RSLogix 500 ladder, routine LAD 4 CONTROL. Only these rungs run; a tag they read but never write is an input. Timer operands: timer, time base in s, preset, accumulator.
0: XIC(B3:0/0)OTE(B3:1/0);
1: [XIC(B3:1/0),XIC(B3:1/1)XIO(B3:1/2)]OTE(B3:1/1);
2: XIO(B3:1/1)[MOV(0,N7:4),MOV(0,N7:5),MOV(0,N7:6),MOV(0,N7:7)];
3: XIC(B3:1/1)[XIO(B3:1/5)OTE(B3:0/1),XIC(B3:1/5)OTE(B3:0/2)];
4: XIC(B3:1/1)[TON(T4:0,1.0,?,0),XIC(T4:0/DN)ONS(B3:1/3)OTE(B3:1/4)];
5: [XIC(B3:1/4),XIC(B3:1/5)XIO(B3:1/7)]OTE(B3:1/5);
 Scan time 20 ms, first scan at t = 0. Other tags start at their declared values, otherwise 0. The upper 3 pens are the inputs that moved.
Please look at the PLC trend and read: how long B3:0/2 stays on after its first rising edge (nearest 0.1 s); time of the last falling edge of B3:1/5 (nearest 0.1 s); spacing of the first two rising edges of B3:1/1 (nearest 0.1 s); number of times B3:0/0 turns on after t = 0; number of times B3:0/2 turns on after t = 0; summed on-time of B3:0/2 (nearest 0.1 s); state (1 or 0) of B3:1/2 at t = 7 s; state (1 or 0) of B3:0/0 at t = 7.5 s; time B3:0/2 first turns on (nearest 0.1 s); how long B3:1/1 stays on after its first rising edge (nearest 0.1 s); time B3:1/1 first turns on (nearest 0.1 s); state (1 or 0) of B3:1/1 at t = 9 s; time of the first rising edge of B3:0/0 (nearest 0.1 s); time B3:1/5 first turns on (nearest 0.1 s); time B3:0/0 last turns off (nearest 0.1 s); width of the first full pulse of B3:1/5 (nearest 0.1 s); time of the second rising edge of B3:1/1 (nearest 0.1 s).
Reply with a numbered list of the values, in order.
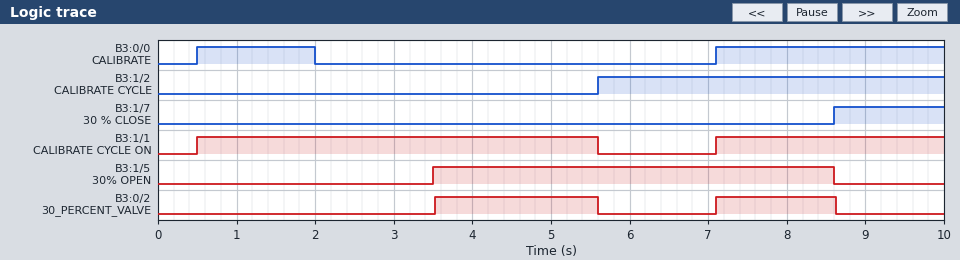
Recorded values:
1. 2.1 s
2. 8.6 s
3. 6.6 s
4. 2
5. 2
6. 3.6 s
7. 1
8. 1
9. 3.5 s
10. 5.1 s
11. 0.5 s
12. 1
13. 0.5 s
14. 3.5 s
15. 2.0 s
16. 5.1 s
17. 7.1 s
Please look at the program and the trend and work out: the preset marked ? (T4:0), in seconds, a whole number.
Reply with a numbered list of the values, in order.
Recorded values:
1. 3 s
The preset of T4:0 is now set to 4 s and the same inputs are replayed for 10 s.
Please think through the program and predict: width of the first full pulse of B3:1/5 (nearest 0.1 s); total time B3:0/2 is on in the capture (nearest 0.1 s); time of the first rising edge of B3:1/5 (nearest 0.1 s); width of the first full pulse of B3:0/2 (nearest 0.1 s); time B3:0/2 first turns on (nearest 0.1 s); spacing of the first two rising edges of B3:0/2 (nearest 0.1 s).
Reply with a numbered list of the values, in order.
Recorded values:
1. 4.1 s
2. 2.6 s
3. 4.5 s
4. 1.1 s
5. 4.5 s
6. 2.6 s
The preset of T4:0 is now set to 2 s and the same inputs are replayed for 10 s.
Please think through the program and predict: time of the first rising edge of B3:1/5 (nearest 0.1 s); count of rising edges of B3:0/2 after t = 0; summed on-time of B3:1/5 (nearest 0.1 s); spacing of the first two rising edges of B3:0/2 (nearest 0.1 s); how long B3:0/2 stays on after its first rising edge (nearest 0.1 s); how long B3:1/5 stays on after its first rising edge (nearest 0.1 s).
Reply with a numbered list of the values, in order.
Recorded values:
1. 2.5 s
2. 3
3. 6.1 s
4. 4.6 s
5. 3.1 s
6. 6.1 s
